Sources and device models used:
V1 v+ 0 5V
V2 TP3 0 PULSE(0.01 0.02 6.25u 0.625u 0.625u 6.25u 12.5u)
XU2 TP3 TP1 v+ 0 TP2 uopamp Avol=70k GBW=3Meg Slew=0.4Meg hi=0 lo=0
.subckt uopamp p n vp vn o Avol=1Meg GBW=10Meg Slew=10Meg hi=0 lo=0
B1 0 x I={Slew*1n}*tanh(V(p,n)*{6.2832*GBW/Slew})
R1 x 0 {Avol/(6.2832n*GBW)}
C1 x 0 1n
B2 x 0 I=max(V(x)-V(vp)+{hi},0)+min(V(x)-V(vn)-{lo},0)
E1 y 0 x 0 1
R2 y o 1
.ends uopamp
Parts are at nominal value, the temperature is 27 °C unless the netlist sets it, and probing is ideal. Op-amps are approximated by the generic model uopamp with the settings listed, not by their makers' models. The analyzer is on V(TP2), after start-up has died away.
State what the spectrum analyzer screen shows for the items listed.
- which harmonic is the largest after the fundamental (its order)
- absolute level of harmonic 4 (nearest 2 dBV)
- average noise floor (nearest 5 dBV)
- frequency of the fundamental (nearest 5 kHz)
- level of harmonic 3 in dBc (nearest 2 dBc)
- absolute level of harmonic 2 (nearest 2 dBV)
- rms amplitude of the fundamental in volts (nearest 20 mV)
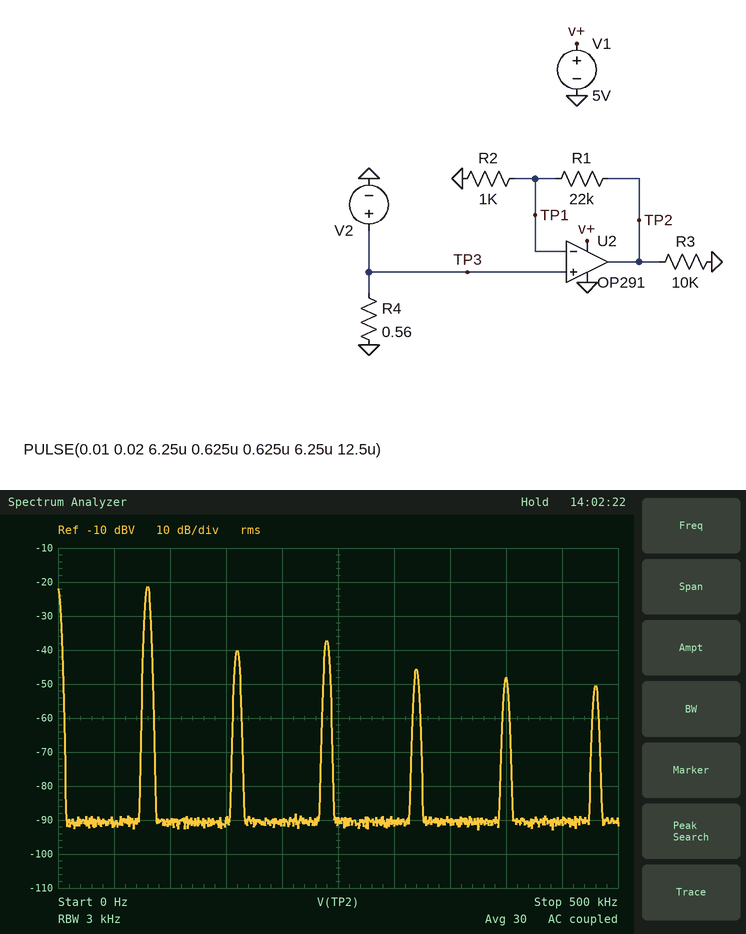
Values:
3
-46 dBV
-90 dBV
80 kHz
-16 dBc
-40 dBV
80 mV
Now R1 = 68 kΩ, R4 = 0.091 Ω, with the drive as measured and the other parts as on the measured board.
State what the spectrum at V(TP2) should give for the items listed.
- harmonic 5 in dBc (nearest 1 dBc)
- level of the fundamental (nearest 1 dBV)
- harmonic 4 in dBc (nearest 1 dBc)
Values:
-31 dBc
-17 dBV
-28 dBc
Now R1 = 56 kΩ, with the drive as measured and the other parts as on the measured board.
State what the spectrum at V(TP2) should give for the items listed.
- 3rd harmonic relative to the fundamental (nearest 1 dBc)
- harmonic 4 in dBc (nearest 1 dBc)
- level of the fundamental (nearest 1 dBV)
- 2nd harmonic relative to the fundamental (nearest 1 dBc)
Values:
-19 dBc
-28 dBc
-17 dBV
-21 dBc
